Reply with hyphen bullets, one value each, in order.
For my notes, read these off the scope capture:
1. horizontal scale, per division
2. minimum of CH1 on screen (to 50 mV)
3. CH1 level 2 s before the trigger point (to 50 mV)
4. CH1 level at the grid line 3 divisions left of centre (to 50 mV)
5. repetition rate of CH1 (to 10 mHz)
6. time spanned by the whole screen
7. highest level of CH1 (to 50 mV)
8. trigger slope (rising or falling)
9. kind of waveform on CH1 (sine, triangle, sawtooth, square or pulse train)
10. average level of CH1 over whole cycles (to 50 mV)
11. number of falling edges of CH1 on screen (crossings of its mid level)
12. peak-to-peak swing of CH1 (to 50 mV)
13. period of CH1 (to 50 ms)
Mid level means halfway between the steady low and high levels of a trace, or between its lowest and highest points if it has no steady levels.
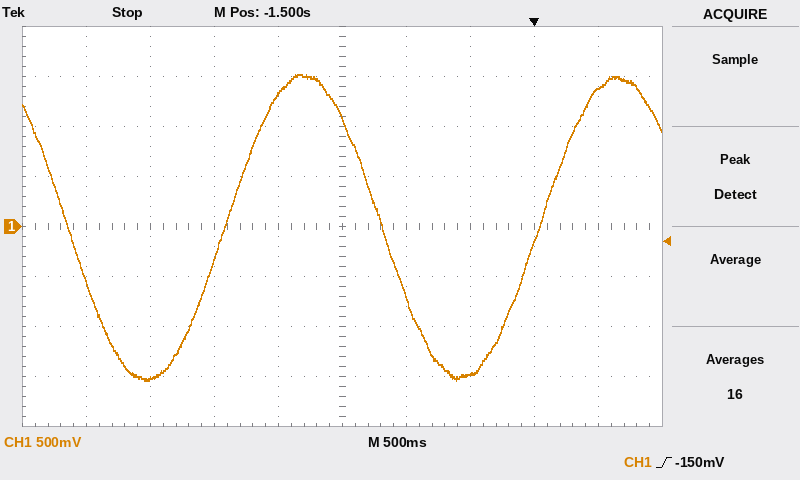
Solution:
- 500 ms
- -1.55 V
- 1.30 V
- -1.50 V
- 410 mHz
- 5 s
- 1.50 V
- rising
- sine
- 0 mV
- 2
- 3.05 V
- 2.45 s
